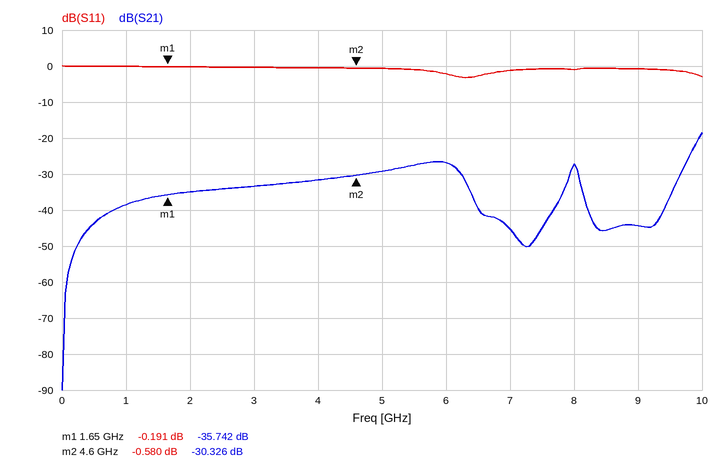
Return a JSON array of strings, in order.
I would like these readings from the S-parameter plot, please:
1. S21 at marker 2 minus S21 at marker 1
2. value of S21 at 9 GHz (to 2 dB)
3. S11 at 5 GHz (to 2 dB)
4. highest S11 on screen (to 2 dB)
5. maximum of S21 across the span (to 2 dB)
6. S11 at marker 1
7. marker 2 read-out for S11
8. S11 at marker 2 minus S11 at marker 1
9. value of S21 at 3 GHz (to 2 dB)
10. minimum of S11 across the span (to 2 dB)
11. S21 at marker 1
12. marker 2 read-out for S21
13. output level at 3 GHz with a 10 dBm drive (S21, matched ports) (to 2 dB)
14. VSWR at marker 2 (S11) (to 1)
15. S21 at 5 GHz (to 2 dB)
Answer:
["5.416 dB", "-44 dB", "0 dB", "0 dB", "-18 dB", "-0.191 dB", "-0.580 dB", "-0.389 dB", "-34 dB", "-4 dB", "-35.742 dB", "-30.326 dB", "-24 dBm", "30", "-30 dB"]
